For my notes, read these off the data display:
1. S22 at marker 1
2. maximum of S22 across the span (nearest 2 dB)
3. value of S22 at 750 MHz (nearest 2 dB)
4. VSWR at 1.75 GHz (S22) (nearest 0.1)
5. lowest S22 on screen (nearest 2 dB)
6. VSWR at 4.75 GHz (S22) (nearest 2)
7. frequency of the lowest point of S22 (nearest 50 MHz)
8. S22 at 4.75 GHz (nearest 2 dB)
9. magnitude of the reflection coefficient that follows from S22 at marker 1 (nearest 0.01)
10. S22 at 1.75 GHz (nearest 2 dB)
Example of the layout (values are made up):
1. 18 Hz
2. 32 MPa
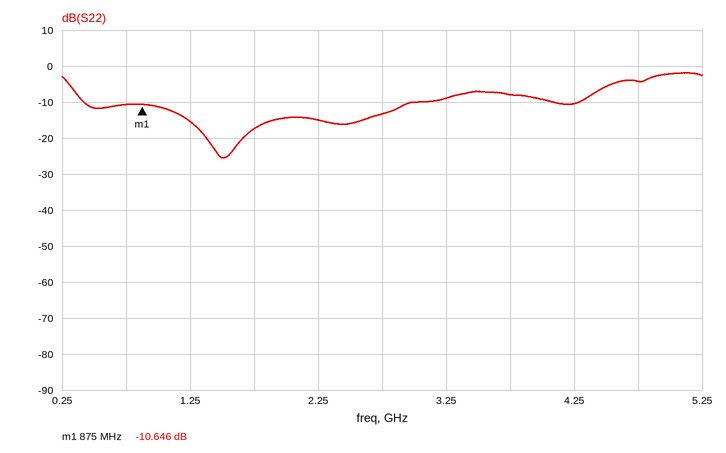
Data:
1. -10.646 dB
2. -2 dB
3. -10 dB
4. 1.3
5. -26 dB
6. 4
7. 1.50 GHz
8. -4 dB
9. 0.29
10. -18 dB
